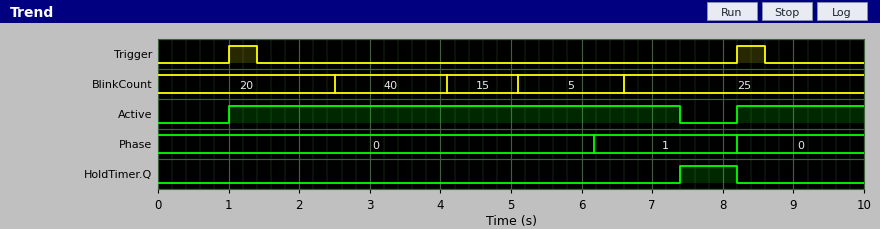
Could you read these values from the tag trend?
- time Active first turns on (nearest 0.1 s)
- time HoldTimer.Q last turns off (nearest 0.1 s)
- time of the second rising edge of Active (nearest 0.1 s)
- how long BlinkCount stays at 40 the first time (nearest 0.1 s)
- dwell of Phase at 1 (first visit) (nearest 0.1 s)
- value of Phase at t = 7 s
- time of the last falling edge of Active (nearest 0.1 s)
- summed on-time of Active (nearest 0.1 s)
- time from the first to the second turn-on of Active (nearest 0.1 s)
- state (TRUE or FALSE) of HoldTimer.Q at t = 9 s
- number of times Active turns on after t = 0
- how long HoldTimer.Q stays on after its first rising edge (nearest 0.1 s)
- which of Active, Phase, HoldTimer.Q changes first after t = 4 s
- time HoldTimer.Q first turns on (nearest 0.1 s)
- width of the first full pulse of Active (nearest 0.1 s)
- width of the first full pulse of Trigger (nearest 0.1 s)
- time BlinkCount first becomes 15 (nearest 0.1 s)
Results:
1.0 s
8.2 s
8.2 s
1.6 s
2.0 s
1
7.4 s
8.2 s
7.2 s
FALSE
2
0.8 s
Phase
7.4 s
6.4 s
0.4 s
4.1 s
